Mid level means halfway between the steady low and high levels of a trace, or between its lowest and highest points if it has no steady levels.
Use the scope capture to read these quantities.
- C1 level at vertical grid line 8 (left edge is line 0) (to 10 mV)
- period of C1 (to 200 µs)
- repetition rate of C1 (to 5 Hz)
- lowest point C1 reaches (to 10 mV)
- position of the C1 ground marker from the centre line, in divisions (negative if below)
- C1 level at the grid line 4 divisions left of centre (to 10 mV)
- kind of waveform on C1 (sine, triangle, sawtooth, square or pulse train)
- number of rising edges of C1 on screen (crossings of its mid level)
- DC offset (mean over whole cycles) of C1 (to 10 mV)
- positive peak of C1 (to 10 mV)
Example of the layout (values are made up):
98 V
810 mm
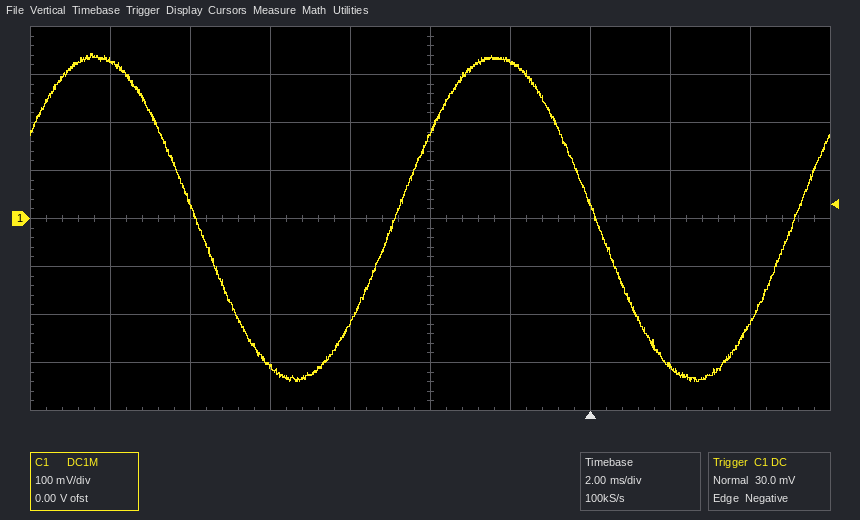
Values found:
-310 mV
10.0 ms
100 Hz
-340 mV
0.0 div
330 mV
sine
2
0 mV
340 mV
